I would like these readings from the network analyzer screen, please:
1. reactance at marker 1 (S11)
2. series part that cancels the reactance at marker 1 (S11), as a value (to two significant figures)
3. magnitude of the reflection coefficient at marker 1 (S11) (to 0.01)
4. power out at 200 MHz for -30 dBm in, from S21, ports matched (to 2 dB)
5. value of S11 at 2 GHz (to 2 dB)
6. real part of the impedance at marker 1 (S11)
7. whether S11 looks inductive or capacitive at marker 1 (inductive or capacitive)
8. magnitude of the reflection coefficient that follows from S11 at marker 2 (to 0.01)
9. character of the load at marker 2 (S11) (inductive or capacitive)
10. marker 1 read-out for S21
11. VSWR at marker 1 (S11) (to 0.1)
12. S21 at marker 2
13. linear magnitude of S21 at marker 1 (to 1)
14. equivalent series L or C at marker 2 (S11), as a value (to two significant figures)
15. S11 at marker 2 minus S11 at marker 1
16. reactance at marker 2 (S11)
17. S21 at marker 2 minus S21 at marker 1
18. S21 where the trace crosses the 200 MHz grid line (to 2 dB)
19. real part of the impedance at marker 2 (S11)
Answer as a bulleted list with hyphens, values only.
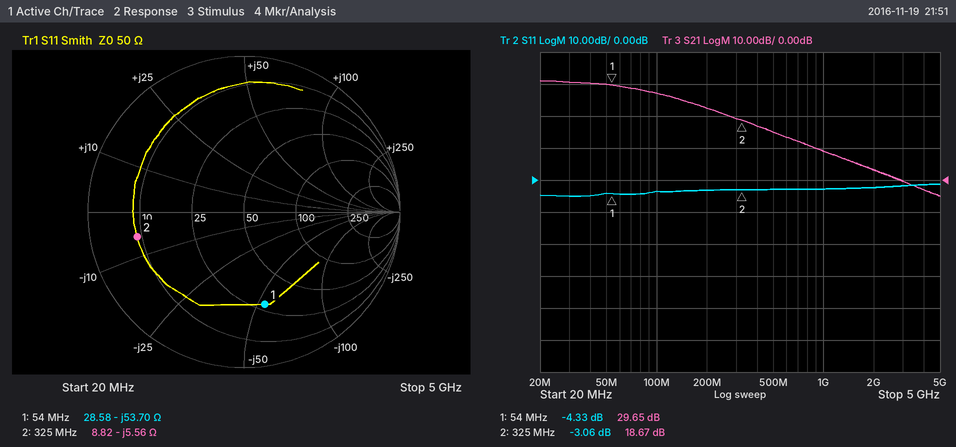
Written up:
- -53.70 Ω
- 160 nH
- 0.61
- -8 dBm
- -2 dB
- 28.58 Ω
- capacitive
- 0.70
- capacitive
- 29.65 dB
- 4.1
- 18.67 dB
- 30
- 88 pF
- 1.27 dB
- -5.56 Ω
- -10.98 dB
- 22 dB
- 8.82 Ω
